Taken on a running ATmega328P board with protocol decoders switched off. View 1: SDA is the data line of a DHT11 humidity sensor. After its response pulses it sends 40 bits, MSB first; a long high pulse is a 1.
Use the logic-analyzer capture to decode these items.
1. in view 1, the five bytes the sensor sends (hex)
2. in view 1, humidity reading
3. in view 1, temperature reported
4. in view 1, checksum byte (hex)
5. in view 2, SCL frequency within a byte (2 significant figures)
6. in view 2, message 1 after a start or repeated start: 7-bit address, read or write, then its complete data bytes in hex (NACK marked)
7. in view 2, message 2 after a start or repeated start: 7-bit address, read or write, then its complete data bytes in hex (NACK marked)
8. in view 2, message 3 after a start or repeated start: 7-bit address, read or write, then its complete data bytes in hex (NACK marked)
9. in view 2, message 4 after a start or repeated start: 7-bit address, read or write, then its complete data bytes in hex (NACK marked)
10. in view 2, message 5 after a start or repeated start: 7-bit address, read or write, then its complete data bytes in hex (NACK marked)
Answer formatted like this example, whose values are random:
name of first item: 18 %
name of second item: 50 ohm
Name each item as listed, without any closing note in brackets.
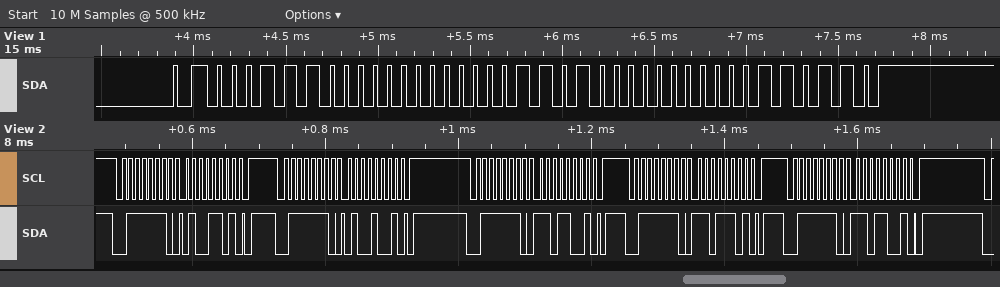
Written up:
in view 1, the five bytes the sensor sends: 1C 00 1A 00 36
in view 1, humidity reading: 28 %
in view 1, temperature reported: 26.0 °C
in view 1, checksum byte: 0x36
in view 2, SCL frequency within a byte: 100 kHz
in view 2, message 1 after a start or repeated start: 7-bit address, read or write, then its complete data bytes in hex: 0x3F write: 4D
in view 2, message 2 after a start or repeated start: 7-bit address, read or write, then its complete data bytes in hex: 0x3F write: 49
in view 2, message 3 after a start or repeated start: 7-bit address, read or write, then its complete data bytes in hex: 0x3F write: D9
in view 2, message 4 after a start or repeated start: 7-bit address, read or write, then its complete data bytes in hex: 0x3F write: DD
in view 2, message 5 after a start or repeated start: 7-bit address, read or write, then its complete data bytes in hex: 0x3F write: D9
